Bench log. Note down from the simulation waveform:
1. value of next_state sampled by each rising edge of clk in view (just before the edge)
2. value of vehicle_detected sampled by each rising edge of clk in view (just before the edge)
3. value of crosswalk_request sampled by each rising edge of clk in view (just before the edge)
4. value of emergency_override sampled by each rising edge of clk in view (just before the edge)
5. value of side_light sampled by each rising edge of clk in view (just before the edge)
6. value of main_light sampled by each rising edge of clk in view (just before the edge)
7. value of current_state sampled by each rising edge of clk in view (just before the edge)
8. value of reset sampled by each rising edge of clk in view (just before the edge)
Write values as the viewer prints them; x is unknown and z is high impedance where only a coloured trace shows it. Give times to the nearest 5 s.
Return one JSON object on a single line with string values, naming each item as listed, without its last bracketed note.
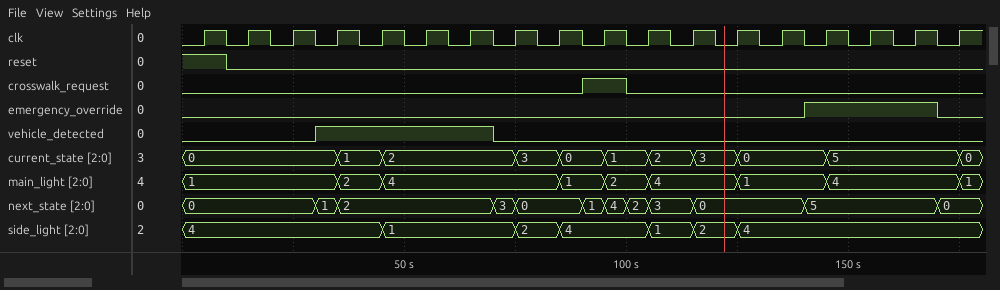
{"value of next_state sampled by each rising edge of clk in view": "0, 0, 0, 1, 2, 2, 2, 3, 0, 1, 2, 3, 0, 0, 5, 5, 5, 0", "value of vehicle_detected sampled by each rising edge of clk in view": "0 0 0 1 1 1 1 0 0 0 0 0 0 0 0 0 0 0", "value of crosswalk_request sampled by each rising edge of clk in view": "0 0 0 0 0 0 0 0 0 1 0 0 0 0 0 0 0 0", "value of emergency_override sampled by each rising edge of clk in view": "0 0 0 0 0 0 0 0 0 0 0 0 0 0 1 1 1 0", "value of side_light sampled by each rising edge of clk in view": "4, 4, 4, 4, 4, 1, 1, 1, 2, 4, 4, 1, 2, 4, 4, 4, 4, 4", "value of main_light sampled by each rising edge of clk in view": "1, 1, 1, 1, 2, 4, 4, 4, 4, 1, 2, 4, 4, 1, 1, 4, 4, 4", "value of current_state sampled by each rising edge of clk in view": "0, 0, 0, 0, 1, 2, 2, 2, 3, 0, 1, 2, 3, 0, 0, 5, 5, 5", "value of reset sampled by each rising edge of clk in view": "1 0 0 0 0 0 0 0 0 0 0 0 0 0 0 0 0 0"}
